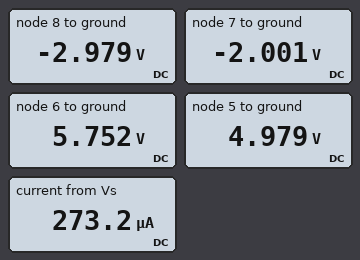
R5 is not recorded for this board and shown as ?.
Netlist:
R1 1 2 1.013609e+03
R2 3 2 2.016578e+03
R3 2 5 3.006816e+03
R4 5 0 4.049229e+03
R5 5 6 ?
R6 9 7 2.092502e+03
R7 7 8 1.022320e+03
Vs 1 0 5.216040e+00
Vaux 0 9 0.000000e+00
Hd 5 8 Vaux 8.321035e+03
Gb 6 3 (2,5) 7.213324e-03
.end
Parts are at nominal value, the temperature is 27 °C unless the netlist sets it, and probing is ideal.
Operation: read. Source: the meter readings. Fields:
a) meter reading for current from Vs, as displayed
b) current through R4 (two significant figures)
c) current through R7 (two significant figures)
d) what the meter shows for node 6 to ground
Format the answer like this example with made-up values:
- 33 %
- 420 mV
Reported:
- 273.2 µA
- 1.2 mA
- 960 µA
- 5.752 V
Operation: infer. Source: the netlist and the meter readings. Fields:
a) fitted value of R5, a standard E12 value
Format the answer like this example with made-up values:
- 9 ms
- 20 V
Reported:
- 2.7 kΩ
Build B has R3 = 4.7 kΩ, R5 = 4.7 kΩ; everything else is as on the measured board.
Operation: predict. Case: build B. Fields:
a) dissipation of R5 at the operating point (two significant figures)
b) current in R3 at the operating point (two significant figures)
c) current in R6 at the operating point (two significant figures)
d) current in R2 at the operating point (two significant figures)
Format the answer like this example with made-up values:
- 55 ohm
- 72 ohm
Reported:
- 370 µW
- 8.3 µA
- 960 µA
- 280 µA
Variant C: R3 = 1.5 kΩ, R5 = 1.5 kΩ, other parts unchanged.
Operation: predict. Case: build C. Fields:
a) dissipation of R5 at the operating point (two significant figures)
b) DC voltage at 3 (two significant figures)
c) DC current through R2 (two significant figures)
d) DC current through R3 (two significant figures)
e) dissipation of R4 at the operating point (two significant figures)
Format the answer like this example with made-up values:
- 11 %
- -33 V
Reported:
- 140 µW
- 4.3 V
- 300 µA
- 28 µA
- 6.1 mW
